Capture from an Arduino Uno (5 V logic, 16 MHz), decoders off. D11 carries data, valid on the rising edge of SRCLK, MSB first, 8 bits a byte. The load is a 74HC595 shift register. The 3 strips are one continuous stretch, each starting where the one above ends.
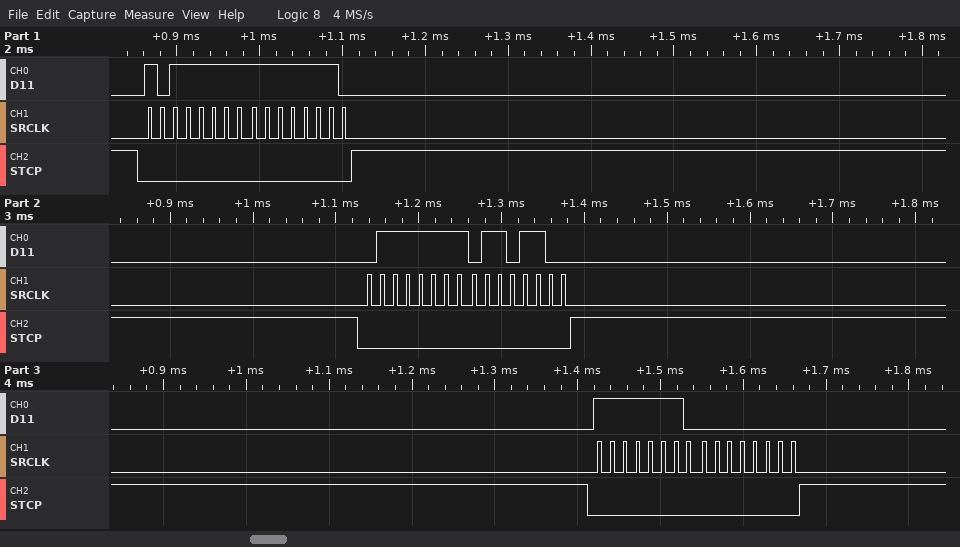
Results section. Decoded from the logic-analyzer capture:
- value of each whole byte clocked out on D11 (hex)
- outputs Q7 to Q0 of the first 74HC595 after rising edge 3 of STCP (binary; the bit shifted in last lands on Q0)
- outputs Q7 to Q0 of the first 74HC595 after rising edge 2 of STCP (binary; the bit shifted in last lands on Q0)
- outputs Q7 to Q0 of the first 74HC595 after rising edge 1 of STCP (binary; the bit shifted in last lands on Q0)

BF FE 7F 6C FE 00
00000000
01101100
11111110
